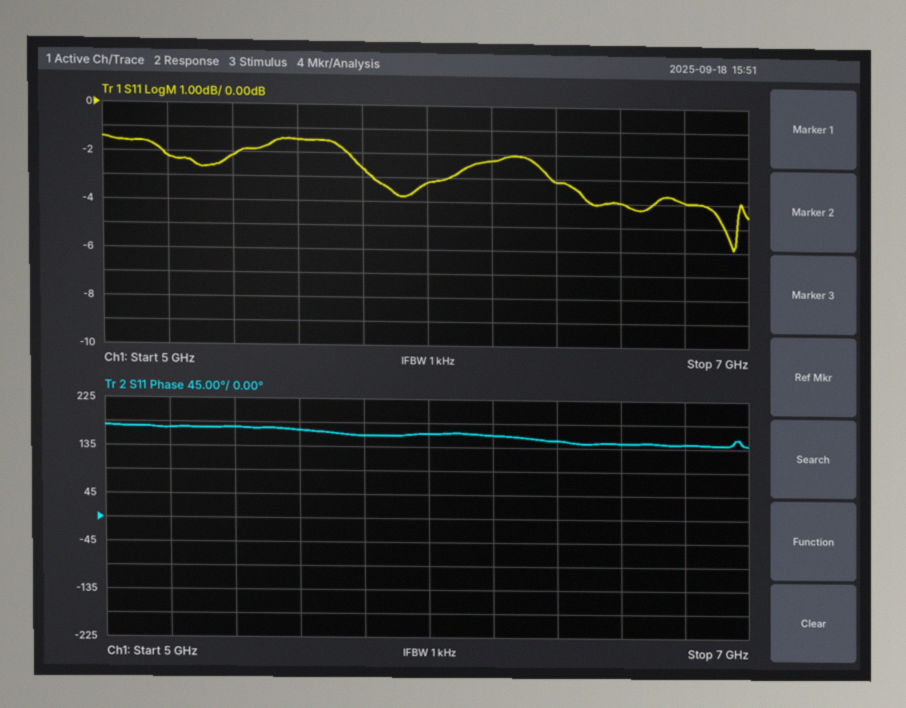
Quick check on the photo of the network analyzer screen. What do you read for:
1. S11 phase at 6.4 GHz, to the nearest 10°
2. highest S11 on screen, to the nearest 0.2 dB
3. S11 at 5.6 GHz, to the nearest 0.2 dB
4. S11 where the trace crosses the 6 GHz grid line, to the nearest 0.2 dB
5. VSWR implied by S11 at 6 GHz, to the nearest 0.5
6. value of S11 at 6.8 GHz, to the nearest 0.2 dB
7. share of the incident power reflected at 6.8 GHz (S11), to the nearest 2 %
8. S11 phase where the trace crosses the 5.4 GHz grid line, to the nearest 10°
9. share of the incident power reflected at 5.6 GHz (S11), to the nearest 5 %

150°
-1.4 dB
-1.4 dB
-3.2 dB
5.5
-4.0 dB
40 %
170°
70 %
